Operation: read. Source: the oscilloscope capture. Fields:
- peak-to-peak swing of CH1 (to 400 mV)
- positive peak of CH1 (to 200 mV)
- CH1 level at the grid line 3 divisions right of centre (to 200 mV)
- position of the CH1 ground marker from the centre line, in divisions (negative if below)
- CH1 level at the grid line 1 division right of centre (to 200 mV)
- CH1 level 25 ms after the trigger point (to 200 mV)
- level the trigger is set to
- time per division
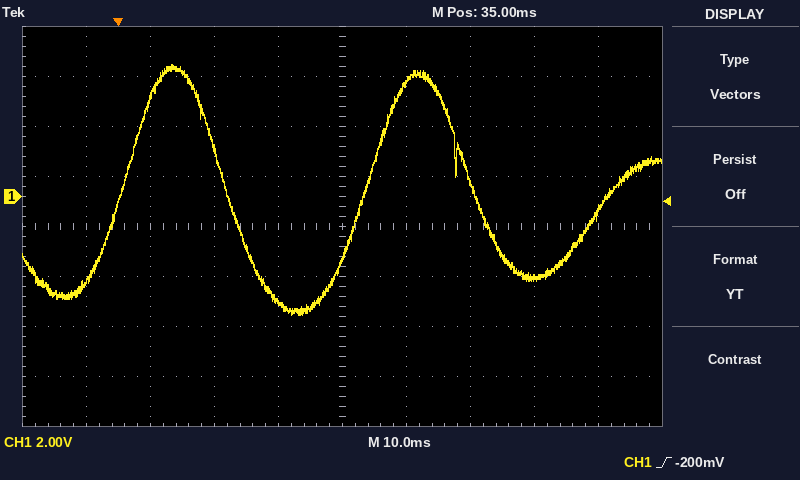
10.0 V
5.2 V
-3.2 V
+0.6 div
4.6 V
-4.2 V
-200 mV
10 ms
